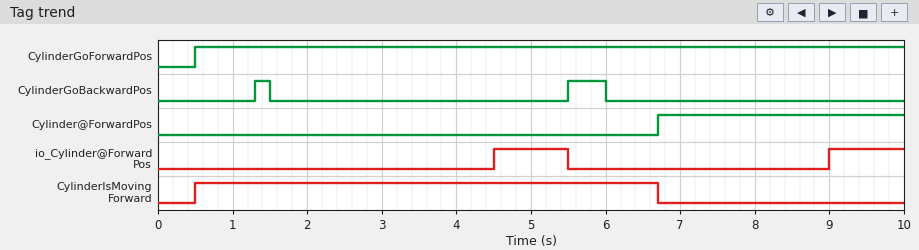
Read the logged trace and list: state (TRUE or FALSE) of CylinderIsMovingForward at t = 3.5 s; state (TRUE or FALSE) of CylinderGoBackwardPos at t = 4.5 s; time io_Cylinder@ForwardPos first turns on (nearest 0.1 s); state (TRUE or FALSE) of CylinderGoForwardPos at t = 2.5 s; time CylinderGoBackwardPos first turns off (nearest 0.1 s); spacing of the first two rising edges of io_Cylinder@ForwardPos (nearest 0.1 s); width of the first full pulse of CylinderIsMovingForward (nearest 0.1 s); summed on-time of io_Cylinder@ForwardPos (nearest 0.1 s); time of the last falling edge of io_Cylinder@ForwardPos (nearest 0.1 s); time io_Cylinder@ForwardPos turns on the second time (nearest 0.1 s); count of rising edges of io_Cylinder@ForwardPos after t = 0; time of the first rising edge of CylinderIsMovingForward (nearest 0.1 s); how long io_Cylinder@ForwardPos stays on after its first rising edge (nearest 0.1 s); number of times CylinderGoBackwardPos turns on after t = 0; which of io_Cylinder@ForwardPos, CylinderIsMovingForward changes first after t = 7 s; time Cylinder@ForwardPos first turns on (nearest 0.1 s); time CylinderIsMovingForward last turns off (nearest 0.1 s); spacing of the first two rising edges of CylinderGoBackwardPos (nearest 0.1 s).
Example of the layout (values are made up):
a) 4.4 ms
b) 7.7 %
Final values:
a) TRUE
b) FALSE
c) 4.5 s
d) TRUE
e) 1.5 s
f) 4.5 s
g) 6.2 s
h) 2.0 s
i) 5.5 s
j) 9.0 s
k) 2
l) 0.5 s
m) 1.0 s
n) 2
o) io_Cylinder@ForwardPos
p) 6.7 s
q) 6.7 s
r) 4.2 s
